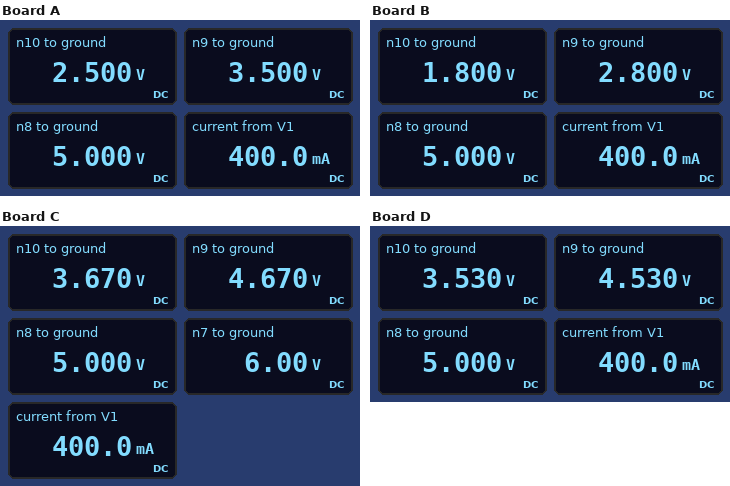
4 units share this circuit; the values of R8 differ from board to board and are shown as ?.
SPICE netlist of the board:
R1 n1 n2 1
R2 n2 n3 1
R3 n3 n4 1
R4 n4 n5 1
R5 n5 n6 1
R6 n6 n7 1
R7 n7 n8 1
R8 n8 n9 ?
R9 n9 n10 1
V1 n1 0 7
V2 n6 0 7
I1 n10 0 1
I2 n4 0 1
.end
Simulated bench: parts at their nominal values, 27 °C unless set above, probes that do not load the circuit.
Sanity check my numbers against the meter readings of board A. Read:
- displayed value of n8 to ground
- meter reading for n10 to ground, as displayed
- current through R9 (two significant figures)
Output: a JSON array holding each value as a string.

["5.000 V", "2.500 V", "1.0 A"]
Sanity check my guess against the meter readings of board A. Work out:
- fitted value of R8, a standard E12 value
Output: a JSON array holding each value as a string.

["1.5 Ω"]
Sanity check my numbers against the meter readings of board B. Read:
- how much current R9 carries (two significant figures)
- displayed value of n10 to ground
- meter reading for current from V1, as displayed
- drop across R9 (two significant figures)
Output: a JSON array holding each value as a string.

["1.0 A", "1.800 V", "400.0 mA", "1.0 V"]
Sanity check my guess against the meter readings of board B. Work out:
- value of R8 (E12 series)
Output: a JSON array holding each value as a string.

["2.2 Ω"]
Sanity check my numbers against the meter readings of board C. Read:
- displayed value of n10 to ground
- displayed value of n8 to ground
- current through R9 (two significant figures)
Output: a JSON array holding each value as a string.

["3.670 V", "5.000 V", "1.0 A"]
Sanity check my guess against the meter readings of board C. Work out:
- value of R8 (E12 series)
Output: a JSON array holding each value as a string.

["0.33 Ω"]
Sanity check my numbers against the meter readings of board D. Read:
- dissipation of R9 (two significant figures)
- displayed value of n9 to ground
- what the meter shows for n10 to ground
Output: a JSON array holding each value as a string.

["1.0 W", "4.530 V", "3.530 V"]
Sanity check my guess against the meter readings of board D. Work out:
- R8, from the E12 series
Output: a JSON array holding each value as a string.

["0.47 Ω"]
